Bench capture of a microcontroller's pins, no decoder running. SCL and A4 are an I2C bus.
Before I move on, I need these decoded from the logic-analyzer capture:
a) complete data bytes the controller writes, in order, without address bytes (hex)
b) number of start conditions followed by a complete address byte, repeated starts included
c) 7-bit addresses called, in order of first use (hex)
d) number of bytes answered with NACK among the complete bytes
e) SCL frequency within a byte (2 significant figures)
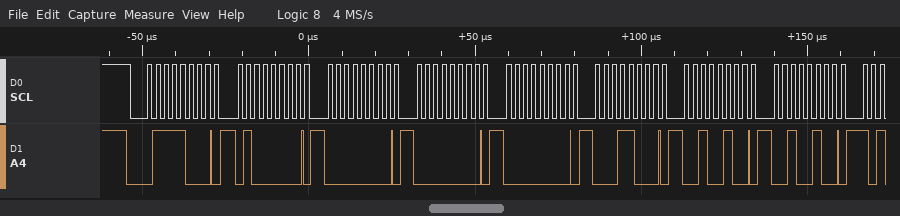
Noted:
40 00 00 00 18 24 24
1
0x3C
0
400 kHz
